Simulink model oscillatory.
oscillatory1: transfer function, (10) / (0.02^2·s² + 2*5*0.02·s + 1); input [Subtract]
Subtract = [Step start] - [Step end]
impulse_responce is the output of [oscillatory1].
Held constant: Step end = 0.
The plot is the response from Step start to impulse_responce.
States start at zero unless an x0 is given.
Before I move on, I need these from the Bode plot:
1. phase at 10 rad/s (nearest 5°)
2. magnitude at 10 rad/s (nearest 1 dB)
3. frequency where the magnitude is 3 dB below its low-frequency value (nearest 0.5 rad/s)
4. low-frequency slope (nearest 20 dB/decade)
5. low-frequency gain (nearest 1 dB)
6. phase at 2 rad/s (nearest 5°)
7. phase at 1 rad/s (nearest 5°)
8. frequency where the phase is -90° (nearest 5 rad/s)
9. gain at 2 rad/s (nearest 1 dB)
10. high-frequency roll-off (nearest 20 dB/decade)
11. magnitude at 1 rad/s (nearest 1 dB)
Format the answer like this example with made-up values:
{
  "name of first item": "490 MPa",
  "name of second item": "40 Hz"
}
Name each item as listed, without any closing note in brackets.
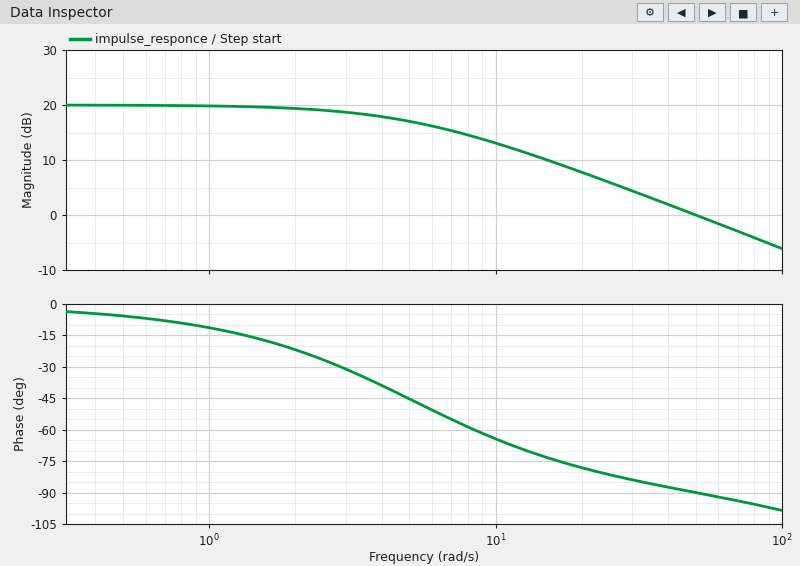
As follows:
{
  "phase at 10 rad/s": "-65°",
  "magnitude at 10 rad/s": "13 dB",
  "frequency where the magnitude is 3 dB below its low-frequency value": "5.0 rad/s",
  "low-frequency slope": "0 dB/decade",
  "low-frequency gain": "20 dB",
  "phase at 2 rad/s": "-20°",
  "phase at 1 rad/s": "-10°",
  "frequency where the phase is -90°": "50 rad/s",
  "gain at 2 rad/s": "19 dB",
  "high-frequency roll-off": "-20 dB/decade",
  "magnitude at 1 rad/s": "20 dB"
}
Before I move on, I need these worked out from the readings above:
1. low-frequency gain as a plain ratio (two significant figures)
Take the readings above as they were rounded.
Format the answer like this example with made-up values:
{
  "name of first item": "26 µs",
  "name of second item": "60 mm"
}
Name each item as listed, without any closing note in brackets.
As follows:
{
  "low-frequency gain as a plain ratio": "10"
}
